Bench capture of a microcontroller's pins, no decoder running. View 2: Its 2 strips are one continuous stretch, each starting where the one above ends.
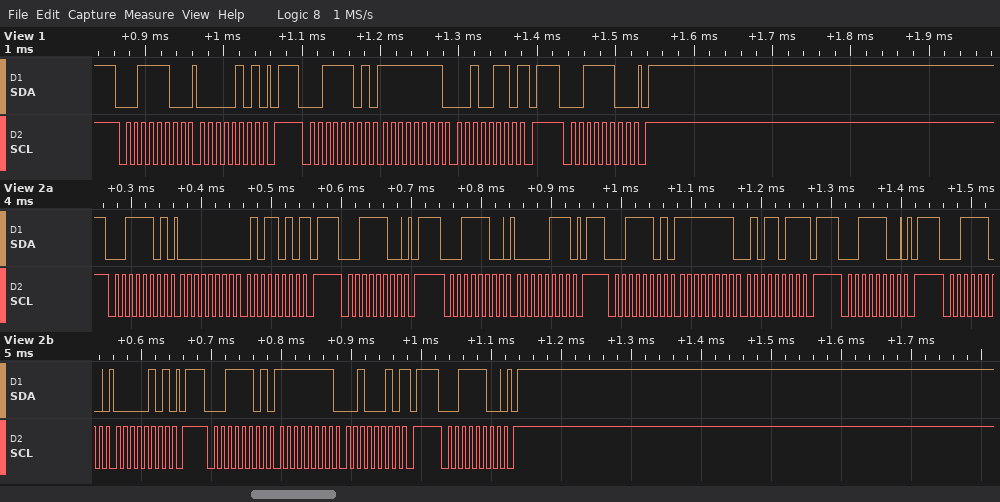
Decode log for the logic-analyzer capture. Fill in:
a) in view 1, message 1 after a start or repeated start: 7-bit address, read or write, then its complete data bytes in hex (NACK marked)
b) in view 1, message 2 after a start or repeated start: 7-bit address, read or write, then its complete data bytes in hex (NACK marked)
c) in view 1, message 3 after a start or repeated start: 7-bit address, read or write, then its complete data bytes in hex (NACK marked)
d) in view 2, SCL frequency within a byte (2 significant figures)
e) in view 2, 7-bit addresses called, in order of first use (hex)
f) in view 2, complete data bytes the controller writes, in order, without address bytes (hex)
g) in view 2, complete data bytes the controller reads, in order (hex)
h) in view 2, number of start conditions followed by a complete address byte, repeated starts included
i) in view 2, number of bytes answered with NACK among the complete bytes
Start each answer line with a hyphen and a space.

- 0x1E write: 05
- 0x1E read: FF 26 NACK
- 0x1E write
- 100 kHz
- 0x1E
- 07 05
- 00 5A FF 5B FF 22
- 8
- 3
